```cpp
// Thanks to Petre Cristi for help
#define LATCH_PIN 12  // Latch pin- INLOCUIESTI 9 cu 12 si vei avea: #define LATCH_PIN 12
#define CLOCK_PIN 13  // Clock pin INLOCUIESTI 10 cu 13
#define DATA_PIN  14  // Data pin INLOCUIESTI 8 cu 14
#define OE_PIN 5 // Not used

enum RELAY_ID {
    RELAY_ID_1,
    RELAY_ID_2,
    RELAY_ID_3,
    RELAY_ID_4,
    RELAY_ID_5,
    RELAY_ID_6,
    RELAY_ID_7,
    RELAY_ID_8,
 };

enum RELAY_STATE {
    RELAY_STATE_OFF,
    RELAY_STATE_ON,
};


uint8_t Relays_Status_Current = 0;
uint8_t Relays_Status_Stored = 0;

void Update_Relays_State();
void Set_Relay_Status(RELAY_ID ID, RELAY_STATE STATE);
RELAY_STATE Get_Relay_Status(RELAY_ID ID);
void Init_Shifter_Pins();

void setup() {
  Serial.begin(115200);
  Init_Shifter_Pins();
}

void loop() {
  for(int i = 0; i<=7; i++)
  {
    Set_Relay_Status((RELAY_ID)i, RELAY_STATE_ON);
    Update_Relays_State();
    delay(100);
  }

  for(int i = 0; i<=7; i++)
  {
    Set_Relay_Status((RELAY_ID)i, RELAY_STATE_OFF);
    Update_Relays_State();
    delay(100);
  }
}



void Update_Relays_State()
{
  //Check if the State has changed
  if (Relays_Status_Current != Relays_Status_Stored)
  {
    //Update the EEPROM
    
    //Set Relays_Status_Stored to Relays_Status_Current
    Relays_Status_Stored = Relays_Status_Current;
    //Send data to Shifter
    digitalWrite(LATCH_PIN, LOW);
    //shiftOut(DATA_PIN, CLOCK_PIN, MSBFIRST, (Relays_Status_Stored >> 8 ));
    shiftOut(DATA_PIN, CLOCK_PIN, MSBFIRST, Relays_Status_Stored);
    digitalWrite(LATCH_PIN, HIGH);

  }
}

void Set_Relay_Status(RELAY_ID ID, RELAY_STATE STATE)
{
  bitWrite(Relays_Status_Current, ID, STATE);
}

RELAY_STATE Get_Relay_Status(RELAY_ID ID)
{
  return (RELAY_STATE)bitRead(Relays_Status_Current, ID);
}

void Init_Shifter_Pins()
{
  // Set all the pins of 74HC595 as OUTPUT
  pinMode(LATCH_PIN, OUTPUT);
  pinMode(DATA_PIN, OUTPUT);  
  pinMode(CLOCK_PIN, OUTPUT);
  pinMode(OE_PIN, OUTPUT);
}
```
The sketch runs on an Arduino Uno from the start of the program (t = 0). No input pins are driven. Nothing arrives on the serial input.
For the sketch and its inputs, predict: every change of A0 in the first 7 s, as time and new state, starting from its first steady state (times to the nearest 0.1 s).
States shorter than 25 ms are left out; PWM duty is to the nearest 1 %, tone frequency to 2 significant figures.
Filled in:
0 s high; 0.8 s low; 1.6 s high; 2.4 s low; 3.2 s high; 4 s low; 4.8 s high; 5.6 s low; 6.4 s high
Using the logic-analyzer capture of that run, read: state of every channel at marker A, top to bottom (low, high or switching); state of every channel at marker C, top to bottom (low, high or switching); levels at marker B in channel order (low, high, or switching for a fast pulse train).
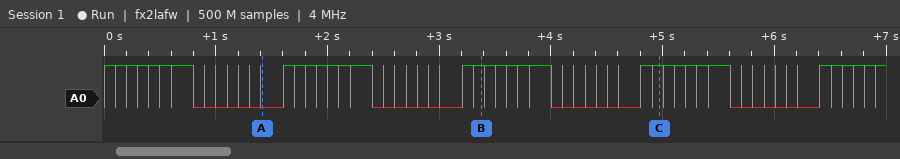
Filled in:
A0 low
A0 high
A0 high
